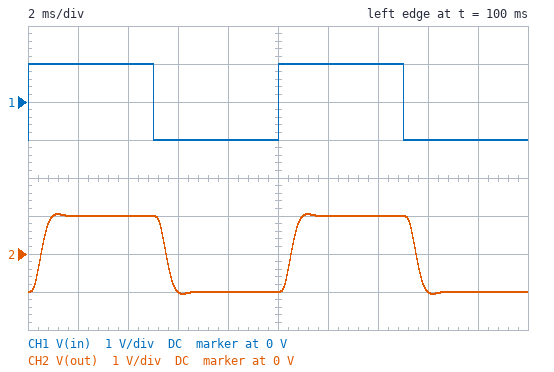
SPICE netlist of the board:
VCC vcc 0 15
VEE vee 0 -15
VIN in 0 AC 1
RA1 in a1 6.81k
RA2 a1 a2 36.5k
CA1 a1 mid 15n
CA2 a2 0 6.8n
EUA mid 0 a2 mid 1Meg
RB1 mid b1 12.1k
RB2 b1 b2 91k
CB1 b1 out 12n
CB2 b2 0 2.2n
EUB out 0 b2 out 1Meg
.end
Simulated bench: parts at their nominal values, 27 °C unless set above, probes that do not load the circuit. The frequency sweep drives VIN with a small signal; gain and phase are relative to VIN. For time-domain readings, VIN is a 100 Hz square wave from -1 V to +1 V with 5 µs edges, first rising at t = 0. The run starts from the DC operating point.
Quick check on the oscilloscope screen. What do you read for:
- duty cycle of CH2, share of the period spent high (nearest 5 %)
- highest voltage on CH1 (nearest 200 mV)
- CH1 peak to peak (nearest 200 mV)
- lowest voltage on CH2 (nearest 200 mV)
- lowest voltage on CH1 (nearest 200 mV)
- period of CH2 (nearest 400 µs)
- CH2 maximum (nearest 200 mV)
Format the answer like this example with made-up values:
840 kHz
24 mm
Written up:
50 %
1.0 V
2.0 V
-1.0 V
-1.0 V
10.0 ms
1.0 V
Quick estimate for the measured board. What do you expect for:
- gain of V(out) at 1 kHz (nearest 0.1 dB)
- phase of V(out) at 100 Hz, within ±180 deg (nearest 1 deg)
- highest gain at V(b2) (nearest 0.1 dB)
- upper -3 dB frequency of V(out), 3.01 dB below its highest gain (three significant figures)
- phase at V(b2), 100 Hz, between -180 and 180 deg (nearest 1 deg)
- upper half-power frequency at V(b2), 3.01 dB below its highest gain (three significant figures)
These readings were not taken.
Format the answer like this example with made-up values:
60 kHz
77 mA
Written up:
-8.5 dB
-19 deg
0 dB
650 Hz
-19 deg
650 Hz
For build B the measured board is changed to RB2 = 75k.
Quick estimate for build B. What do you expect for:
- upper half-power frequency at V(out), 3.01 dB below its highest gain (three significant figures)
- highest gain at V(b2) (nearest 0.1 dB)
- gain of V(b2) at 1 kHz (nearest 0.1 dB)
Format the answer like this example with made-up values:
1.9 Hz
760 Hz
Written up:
714 Hz
0 dB
-7.0 dB
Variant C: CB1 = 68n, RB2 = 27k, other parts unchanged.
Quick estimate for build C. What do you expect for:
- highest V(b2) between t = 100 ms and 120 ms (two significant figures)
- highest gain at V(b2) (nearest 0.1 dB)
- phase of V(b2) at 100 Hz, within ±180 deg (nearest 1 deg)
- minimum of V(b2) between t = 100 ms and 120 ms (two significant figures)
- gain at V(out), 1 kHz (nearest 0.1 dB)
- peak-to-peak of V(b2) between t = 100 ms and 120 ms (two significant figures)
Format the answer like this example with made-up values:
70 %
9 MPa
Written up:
1.7 V
5.6 dB
-14 deg
-1.7 V
-6.0 dB
3.5 V
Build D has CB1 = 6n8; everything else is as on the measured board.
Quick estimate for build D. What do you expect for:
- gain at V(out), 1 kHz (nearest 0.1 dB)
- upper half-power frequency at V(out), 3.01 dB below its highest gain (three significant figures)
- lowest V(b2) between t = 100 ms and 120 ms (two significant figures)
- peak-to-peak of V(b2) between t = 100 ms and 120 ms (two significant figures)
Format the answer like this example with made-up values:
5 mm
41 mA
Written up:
-8.7 dB
568 Hz
-1.0 V
2.0 V
